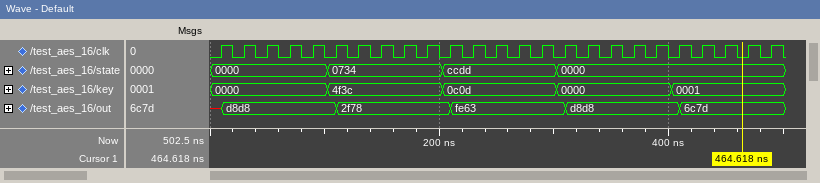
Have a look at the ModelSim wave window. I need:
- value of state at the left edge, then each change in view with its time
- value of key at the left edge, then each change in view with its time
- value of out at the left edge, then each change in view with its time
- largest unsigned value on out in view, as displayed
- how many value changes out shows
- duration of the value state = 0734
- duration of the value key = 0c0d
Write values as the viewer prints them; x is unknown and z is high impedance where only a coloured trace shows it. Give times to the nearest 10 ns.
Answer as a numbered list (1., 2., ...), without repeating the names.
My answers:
1. 0000, 0734 at 100 ns, ccdd at 200 ns, 0000 at 300 ns
2. 0000, 4f3c at 100 ns, 0c0d at 200 ns, 0000 at 300 ns, 0001 at 400 ns
3. x, d8d8 at 10 ns, 2f78 at 110 ns, fe63 at 210 ns, d8d8 at 310 ns, 6c7d at 410 ns
4. fe63
5. 5
6. 100 ns
7. 100 ns
